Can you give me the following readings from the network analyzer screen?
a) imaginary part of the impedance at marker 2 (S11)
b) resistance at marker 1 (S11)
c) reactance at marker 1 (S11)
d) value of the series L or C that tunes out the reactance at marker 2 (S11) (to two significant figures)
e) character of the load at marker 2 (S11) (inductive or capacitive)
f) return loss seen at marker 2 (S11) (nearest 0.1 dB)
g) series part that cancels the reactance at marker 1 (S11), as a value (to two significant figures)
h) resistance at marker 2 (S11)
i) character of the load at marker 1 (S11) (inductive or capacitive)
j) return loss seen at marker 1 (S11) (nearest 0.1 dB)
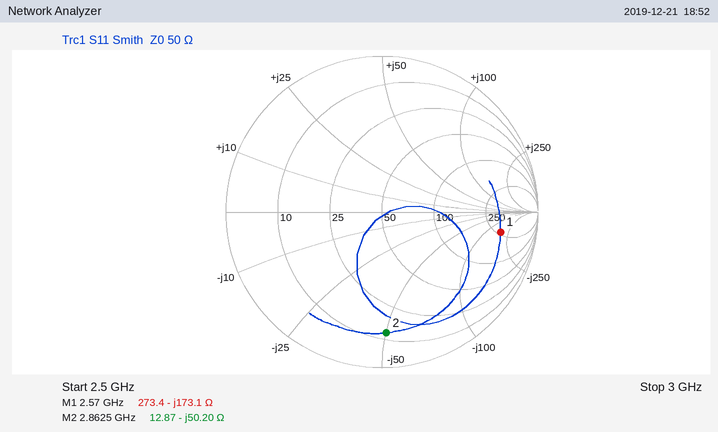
-50.20 Ω
273.4 Ω
-173.1 Ω
2.8 nH
capacitive
2.2 dB
11 nH
12.87 Ω
capacitive
2.3 dB
